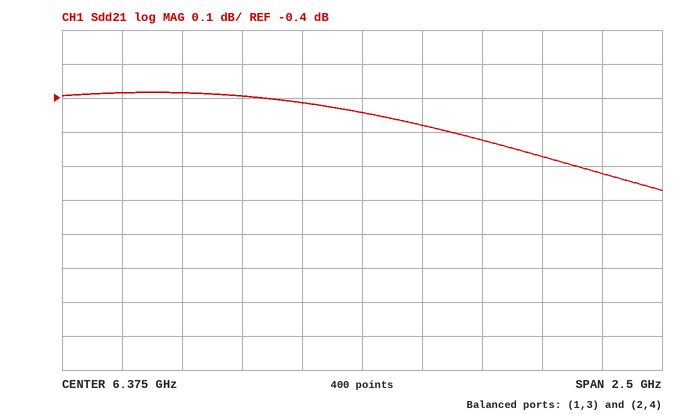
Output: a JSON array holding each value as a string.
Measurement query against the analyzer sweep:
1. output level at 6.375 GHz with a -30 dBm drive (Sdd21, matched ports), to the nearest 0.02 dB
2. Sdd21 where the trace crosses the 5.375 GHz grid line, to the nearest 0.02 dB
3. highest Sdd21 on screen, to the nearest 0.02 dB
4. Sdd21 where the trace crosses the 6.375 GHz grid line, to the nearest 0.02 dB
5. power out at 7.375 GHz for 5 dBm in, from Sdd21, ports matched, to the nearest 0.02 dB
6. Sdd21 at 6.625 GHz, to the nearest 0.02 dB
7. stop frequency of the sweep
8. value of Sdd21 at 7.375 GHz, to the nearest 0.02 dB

["-30.44 dBm", "-0.38 dB", "-0.38 dB", "-0.44 dB", "4.38 dBm", "-0.48 dB", "7.625 GHz", "-0.62 dB"]
